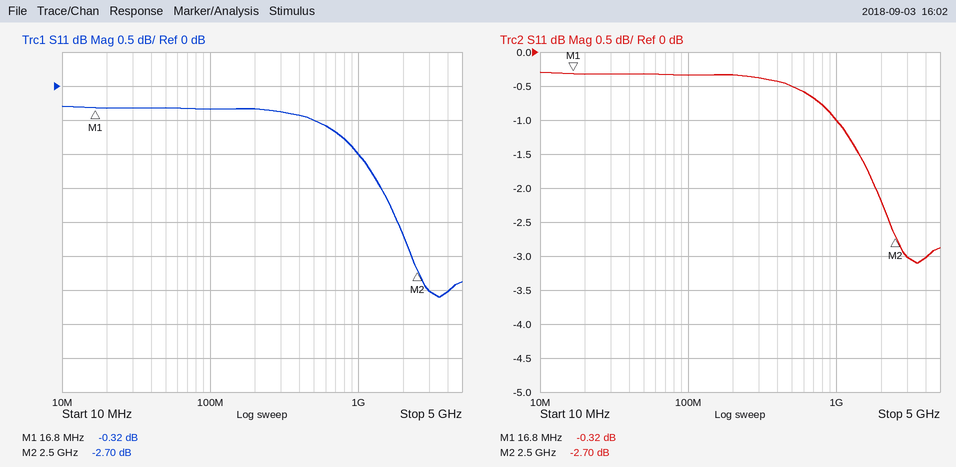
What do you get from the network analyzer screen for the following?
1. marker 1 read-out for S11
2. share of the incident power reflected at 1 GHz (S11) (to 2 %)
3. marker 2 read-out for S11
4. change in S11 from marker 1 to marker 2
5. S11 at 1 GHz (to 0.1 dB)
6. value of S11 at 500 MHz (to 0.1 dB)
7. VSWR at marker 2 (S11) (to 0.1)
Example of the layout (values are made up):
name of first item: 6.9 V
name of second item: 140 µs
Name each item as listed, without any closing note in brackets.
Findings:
marker 1 read-out for S11: -0.32 dB
share of the incident power reflected at 1 GHz (S11): 80 %
marker 2 read-out for S11: -2.70 dB
change in S11 from marker 1 to marker 2: -2.38 dB
S11 at 1 GHz: -1.0 dB
value of S11 at 500 MHz: -0.5 dB
VSWR at marker 2 (S11): 6.5
